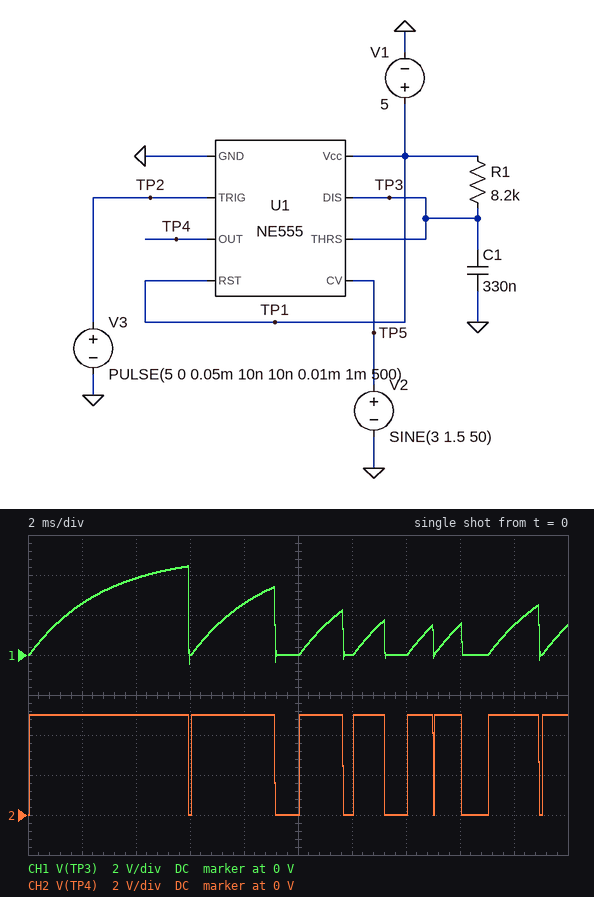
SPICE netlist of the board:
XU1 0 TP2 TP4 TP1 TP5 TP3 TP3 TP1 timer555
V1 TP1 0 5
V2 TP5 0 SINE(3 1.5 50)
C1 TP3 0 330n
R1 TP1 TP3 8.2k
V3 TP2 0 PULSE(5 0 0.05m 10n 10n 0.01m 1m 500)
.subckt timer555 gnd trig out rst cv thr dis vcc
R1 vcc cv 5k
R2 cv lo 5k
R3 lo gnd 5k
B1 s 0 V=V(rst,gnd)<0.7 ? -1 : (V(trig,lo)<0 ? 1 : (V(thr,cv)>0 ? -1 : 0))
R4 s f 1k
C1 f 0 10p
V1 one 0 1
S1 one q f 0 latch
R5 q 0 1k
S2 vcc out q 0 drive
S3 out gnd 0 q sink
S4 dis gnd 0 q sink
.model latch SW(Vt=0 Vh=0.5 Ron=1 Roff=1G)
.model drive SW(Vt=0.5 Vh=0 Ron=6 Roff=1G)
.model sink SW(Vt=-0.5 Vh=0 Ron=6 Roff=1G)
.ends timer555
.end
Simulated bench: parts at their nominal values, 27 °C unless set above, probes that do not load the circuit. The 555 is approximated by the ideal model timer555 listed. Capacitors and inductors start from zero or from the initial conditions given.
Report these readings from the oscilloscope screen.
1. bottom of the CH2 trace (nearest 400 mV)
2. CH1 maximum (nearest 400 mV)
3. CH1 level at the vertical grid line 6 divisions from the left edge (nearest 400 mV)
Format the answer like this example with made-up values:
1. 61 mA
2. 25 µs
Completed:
1. 0 V
2. 4.4 V
3. 0 V
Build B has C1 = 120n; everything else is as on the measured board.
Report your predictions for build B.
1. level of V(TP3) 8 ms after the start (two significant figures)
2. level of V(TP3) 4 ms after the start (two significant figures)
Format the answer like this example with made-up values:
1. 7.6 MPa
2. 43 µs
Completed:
1. 3.1 V
2. 4.3 V
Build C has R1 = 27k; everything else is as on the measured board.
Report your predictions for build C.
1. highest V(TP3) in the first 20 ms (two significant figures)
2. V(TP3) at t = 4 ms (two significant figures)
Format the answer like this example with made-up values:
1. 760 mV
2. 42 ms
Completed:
1. 3.3 V
2. 1.8 V
